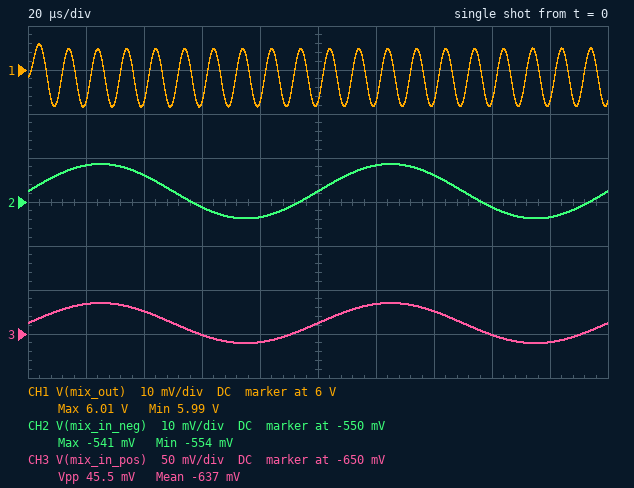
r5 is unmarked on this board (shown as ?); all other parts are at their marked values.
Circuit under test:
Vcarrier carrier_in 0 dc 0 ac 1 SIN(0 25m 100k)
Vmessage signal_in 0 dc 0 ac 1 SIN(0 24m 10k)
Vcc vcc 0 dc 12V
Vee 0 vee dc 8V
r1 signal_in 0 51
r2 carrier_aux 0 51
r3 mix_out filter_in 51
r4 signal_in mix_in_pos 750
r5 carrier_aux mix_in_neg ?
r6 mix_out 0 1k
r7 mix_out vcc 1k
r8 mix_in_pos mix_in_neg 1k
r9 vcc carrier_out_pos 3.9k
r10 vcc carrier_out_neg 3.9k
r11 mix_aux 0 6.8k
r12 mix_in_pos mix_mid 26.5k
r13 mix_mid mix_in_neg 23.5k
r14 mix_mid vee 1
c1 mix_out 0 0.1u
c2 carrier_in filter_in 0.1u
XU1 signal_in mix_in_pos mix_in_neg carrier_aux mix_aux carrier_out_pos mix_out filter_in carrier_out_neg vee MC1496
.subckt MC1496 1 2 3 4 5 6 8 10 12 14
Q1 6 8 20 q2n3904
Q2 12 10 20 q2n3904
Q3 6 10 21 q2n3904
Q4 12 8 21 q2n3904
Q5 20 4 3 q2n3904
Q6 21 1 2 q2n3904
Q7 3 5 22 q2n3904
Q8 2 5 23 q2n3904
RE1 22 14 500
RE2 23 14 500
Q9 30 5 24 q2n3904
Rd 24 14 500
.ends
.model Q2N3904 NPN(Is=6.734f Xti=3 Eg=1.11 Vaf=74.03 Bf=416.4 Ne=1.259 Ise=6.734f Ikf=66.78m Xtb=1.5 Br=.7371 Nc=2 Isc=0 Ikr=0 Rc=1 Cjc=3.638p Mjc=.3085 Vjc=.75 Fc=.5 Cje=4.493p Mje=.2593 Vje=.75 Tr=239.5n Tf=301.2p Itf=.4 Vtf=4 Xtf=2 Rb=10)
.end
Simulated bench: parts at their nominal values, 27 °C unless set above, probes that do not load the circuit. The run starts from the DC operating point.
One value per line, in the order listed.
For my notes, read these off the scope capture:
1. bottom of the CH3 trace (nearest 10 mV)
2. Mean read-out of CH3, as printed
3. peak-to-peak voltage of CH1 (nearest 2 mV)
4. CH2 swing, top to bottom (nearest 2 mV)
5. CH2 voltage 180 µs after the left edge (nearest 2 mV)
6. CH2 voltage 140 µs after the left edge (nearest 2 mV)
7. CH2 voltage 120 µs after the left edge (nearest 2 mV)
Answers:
-660 mV
-637 mV
14 mV
12 mV
-554 mV
-544 mV
-542 mV
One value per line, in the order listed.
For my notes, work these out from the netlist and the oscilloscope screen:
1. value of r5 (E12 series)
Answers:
330 Ω
